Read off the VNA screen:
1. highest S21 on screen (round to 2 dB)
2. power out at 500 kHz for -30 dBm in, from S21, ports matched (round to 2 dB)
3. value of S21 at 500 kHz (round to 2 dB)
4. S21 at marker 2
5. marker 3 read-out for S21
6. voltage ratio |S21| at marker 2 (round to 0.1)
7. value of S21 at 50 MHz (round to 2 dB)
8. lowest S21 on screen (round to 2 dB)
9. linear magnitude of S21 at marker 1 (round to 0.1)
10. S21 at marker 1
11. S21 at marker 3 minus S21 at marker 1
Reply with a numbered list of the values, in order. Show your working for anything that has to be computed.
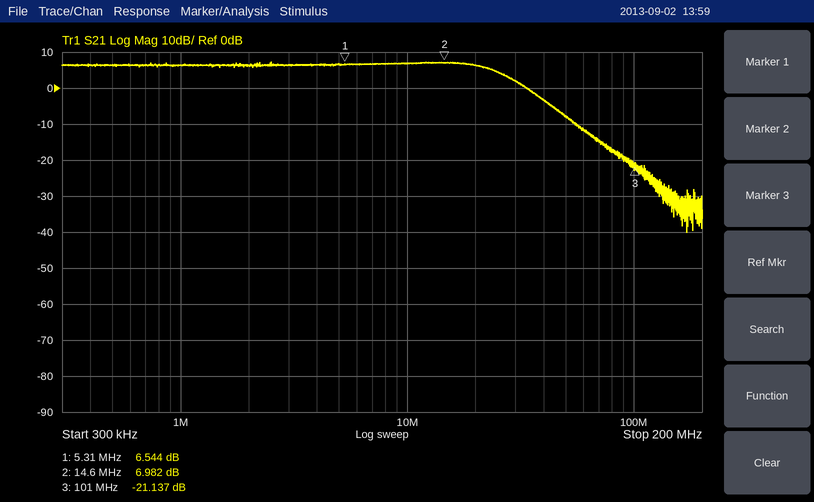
1. 8 dB
2. -30 dBm + (6 dB) = -24 dBm
3. 6 dB
4. 6.982 dB
5. -21.137 dB
6. 10^(6.982/20) ≈ 2.2
7. -8 dB
8. -40 dB
9. 10^(6.544/20) ≈ 2.1
10. 6.544 dB
11. -21.137 − (6.544) = -27.681 dB
